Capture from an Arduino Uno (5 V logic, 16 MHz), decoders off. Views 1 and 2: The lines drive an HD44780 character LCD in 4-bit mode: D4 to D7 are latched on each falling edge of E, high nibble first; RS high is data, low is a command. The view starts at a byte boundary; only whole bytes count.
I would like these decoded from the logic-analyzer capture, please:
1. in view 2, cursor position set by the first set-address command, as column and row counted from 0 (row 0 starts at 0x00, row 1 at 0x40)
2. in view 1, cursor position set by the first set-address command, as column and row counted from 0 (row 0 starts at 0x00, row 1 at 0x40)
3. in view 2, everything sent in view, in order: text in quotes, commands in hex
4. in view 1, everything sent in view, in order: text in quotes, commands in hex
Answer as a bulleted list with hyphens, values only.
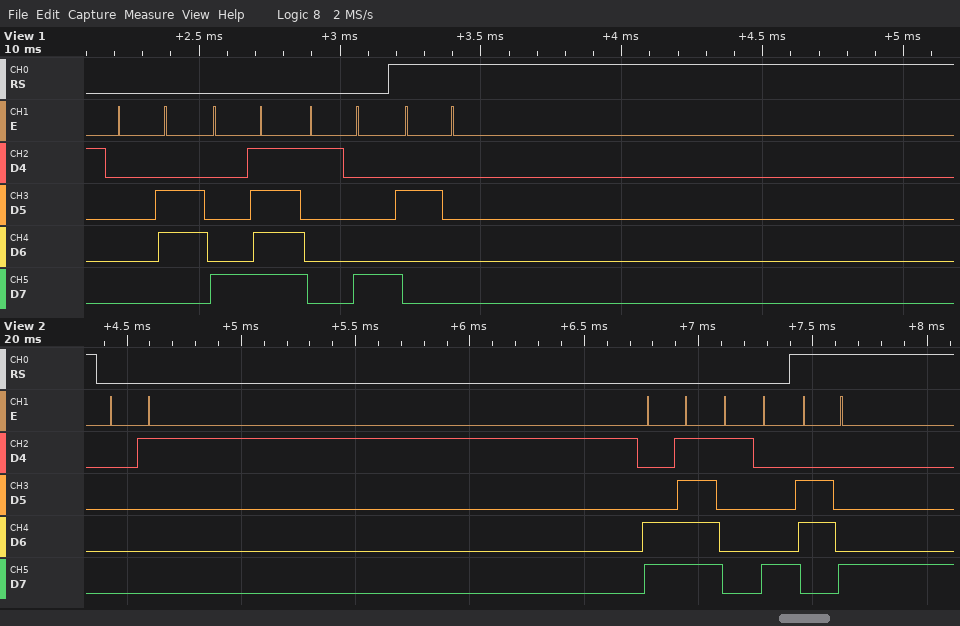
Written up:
- column 15, row 1
- column 15, row 0
- 0x01 0xCF 0x18 "h"
- 0x06 0x8F 0x18 " "
